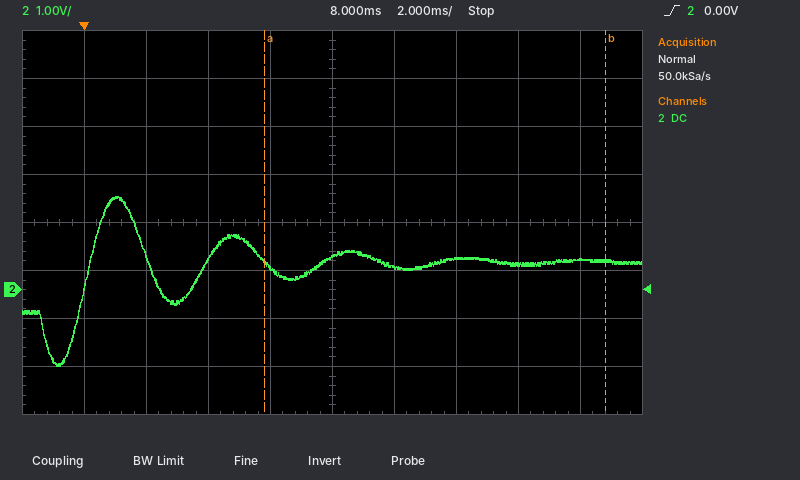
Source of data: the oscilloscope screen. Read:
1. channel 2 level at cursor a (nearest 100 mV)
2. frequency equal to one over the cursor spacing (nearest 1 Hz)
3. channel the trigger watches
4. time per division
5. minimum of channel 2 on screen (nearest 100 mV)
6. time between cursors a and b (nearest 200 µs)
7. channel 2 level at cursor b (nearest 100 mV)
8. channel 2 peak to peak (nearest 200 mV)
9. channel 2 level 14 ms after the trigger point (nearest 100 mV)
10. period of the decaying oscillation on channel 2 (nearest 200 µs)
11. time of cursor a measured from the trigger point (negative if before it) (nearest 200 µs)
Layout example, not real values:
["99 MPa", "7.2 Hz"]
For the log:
["600 mV", "91 Hz", "channel 2", "2 ms", "-1.6 V", "11.0 ms", "600 mV", "3.6 V", "500 mV", "3.8 ms", "+5.8 ms"]
